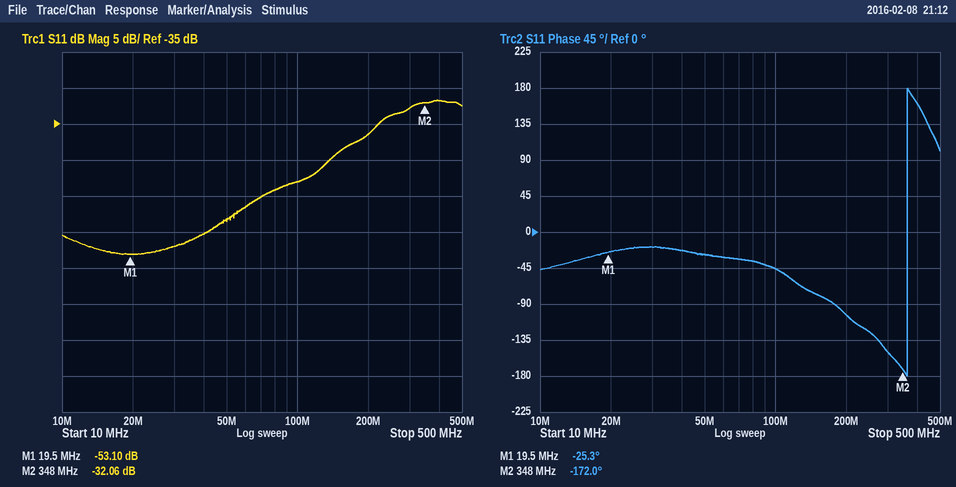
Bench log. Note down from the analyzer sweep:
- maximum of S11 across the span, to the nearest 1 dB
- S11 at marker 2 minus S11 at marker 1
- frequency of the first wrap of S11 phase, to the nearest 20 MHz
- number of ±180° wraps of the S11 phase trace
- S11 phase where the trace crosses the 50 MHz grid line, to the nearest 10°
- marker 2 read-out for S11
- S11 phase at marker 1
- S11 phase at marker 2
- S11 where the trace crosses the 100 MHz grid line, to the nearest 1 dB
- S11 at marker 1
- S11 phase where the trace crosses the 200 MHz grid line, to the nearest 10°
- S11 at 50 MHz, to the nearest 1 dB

-32 dB
21.04 dB
360 MHz
1
-30°
-32.06 dB
-25.3°
-172.0°
-43 dB
-53.10 dB
-100°
-48 dB
